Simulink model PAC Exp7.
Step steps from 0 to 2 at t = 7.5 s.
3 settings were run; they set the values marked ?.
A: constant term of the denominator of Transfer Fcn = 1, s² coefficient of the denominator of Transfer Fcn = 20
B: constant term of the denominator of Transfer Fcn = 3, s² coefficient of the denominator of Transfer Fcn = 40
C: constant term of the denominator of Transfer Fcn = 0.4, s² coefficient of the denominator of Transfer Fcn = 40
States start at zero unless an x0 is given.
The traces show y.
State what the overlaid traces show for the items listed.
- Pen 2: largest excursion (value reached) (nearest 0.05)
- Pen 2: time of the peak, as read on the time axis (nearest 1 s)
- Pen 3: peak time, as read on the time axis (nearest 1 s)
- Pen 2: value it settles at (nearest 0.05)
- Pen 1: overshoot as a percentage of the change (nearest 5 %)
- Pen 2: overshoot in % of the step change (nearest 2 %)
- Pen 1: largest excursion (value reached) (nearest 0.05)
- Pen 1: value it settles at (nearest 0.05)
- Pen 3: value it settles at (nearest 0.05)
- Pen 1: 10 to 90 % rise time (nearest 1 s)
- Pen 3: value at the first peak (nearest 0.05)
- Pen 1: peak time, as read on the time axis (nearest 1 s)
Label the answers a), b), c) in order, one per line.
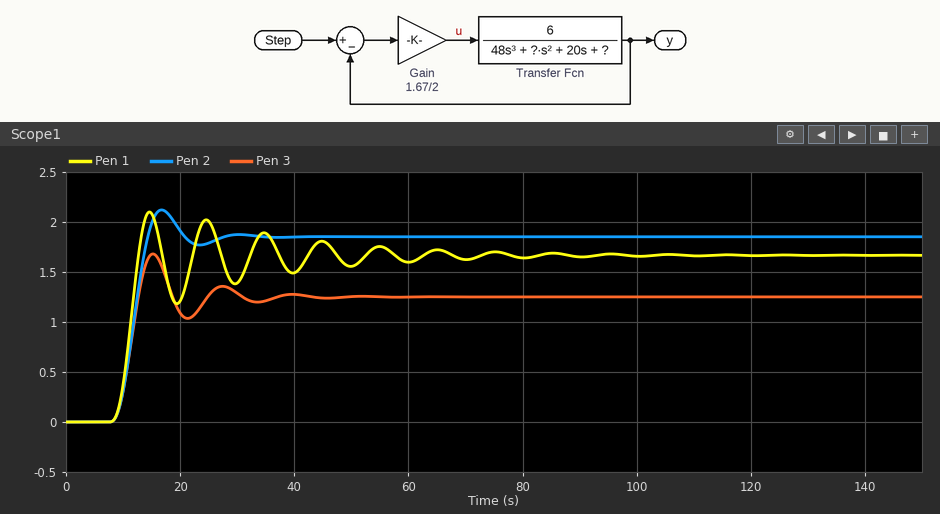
a) 2.10
b) 17 s
c) 15 s
d) 1.85
e) 25 %
f) 14 %
g) 2.10
h) 1.65
i) 1.25
j) 3 s
k) 1.70
l) 15 s
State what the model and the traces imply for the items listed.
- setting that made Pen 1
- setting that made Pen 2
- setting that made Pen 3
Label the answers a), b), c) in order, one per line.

a) A
b) C
c) B
